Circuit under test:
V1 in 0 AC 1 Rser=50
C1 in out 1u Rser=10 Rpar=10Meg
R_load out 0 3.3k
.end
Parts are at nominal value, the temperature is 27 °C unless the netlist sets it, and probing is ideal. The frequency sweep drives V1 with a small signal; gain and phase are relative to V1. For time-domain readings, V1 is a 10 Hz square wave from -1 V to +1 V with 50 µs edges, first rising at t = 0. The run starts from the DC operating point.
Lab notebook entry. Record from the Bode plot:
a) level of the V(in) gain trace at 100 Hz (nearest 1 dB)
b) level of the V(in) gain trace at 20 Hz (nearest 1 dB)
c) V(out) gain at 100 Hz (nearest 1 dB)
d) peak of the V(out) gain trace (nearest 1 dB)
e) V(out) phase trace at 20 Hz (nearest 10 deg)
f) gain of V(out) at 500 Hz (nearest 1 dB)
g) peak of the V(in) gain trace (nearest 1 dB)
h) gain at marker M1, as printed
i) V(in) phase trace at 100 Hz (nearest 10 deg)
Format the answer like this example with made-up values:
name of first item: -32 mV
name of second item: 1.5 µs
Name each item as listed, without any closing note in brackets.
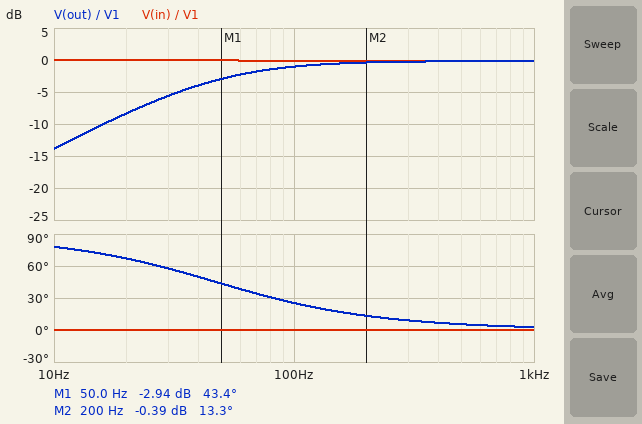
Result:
level of the V(in) gain trace at 100 Hz: 0 dB
level of the V(in) gain trace at 20 Hz: 0 dB
V(out) gain at 100 Hz: -1 dB
peak of the V(out) gain trace: 0 dB
V(out) phase trace at 20 Hz: 70 deg
gain of V(out) at 500 Hz: 0 dB
peak of the V(in) gain trace: 0 dB
gain at marker M1, as printed: -2.94 dB
V(in) phase trace at 100 Hz: 0 deg
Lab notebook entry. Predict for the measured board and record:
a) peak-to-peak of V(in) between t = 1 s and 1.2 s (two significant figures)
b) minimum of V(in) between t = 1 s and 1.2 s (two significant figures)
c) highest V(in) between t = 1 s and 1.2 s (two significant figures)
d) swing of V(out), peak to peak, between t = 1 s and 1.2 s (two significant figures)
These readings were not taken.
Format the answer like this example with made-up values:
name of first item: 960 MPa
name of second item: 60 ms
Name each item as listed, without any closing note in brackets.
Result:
peak-to-peak of V(in) between t = 1 s and 1.2 s: 2.0 V
minimum of V(in) between t = 1 s and 1.2 s: -1.0 V
highest V(in) between t = 1 s and 1.2 s: 1.0 V
swing of V(out), peak to peak, between t = 1 s and 1.2 s: 3.9 V
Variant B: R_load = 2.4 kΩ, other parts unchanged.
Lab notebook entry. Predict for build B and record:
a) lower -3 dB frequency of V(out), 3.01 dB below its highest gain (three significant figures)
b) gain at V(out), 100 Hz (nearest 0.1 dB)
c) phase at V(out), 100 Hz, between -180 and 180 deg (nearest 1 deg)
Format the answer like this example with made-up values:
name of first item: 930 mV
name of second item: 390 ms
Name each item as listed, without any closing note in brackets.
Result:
lower -3 dB frequency of V(out), 3.01 dB below its highest gain: 64.7 Hz
gain at V(out), 100 Hz: -1.7 dB
phase at V(out), 100 Hz, between -180 and 180 deg: 33 deg
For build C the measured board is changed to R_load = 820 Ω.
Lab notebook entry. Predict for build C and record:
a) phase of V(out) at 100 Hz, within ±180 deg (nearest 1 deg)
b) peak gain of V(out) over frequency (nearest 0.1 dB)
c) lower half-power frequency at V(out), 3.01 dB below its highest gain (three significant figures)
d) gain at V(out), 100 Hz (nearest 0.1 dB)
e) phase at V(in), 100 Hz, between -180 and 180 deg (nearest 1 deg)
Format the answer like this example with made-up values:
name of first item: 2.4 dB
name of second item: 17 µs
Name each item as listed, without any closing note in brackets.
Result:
phase of V(out) at 100 Hz, within ±180 deg: 61 deg
peak gain of V(out) over frequency: -0.6 dB
lower half-power frequency at V(out), 3.01 dB below its highest gain: 181 Hz
gain at V(out), 100 Hz: -6.9 dB
phase at V(in), 100 Hz, between -180 and 180 deg: -1 deg
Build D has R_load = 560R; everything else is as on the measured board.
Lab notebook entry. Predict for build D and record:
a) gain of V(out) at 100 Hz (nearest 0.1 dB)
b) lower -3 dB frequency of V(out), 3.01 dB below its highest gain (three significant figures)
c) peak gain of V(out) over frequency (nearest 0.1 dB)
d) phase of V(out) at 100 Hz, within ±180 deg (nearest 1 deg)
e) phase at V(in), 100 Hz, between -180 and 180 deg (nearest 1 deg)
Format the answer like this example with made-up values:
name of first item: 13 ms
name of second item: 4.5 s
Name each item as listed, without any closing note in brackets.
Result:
gain of V(out) at 100 Hz: -9.7 dB
lower -3 dB frequency of V(out), 3.01 dB below its highest gain: 257 Hz
peak gain of V(out) over frequency: -0.9 dB
phase of V(out) at 100 Hz, within ±180 deg: 69 deg
phase at V(in), 100 Hz, between -180 and 180 deg: -2 deg
